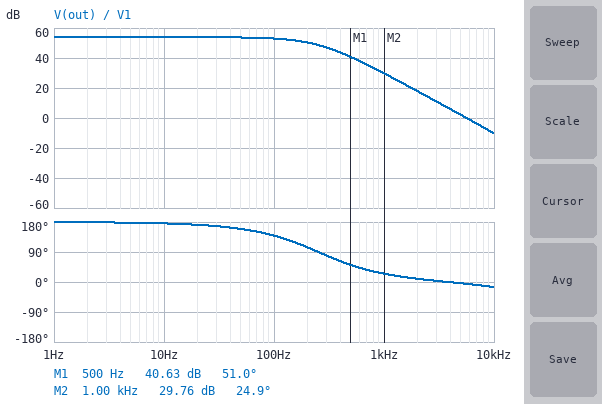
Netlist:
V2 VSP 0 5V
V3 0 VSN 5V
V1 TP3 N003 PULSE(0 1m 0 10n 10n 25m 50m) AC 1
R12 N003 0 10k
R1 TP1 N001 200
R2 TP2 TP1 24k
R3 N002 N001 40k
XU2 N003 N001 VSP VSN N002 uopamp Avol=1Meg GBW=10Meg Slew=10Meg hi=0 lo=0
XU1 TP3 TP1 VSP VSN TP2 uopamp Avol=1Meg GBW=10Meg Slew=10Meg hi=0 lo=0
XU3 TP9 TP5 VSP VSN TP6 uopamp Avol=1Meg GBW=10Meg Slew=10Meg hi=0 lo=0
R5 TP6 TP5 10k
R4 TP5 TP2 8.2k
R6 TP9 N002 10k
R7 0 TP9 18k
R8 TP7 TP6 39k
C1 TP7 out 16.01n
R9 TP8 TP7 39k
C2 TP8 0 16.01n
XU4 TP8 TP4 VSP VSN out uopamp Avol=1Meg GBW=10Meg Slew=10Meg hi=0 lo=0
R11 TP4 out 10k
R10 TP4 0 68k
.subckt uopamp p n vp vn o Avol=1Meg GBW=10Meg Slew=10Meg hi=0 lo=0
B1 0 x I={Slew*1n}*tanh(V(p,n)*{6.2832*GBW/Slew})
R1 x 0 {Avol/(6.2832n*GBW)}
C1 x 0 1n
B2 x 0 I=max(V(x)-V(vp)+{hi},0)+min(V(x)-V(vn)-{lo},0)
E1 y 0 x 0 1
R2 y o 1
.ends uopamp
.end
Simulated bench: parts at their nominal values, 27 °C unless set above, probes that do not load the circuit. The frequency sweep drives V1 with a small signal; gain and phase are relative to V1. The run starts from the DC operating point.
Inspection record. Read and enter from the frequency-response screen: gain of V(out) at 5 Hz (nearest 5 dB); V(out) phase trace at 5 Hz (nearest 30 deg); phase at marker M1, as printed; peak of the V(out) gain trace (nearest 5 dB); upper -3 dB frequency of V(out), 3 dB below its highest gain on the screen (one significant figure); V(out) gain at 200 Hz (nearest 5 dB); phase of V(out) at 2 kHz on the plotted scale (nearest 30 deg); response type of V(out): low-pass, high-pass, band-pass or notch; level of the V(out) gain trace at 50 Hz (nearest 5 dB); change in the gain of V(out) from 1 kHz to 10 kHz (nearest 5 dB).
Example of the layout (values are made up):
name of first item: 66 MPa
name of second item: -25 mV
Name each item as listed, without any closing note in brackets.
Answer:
gain of V(out) at 5 Hz: 55 dB
V(out) phase trace at 5 Hz: 180 deg
phase at marker M1, as printed: 51.0 deg
peak of the V(out) gain trace: 55 dB
upper -3 dB frequency of V(out), 3 dB below its highest gain on the screen: 200 Hz
V(out) gain at 200 Hz: 50 dB
phase of V(out) at 2 kHz on the plotted scale: 0 deg
response type of V(out): low-pass, high-pass, band-pass or notch: low-pass
level of the V(out) gain trace at 50 Hz: 55 dB
change in the gain of V(out) from 1 kHz to 10 kHz: -40 dB
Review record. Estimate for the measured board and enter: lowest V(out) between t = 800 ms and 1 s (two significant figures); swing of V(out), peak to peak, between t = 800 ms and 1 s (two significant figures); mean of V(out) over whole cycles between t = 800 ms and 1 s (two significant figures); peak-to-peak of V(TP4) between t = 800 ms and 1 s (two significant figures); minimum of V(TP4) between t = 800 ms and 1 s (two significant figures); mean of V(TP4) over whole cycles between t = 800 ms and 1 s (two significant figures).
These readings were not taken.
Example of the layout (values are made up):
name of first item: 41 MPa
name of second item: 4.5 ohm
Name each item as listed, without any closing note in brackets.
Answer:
lowest V(out) between t = 800 ms and 1 s: -500 mV
swing of V(out), peak to peak, between t = 800 ms and 1 s: 500 mV
mean of V(out) over whole cycles between t = 800 ms and 1 s: -250 mV
peak-to-peak of V(TP4) between t = 800 ms and 1 s: 430 mV
minimum of V(TP4) between t = 800 ms and 1 s: -430 mV
mean of V(TP4) over whole cycles between t = 800 ms and 1 s: -220 mV
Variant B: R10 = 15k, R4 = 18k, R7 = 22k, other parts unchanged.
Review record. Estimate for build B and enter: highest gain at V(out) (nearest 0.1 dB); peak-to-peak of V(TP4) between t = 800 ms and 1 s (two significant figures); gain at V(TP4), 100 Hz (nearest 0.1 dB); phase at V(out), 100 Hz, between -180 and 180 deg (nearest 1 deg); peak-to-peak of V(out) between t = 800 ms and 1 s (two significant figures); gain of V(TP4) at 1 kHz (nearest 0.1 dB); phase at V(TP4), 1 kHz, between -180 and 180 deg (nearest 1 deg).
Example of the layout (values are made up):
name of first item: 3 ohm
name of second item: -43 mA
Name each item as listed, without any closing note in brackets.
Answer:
highest gain at V(out): 53.5 dB
peak-to-peak of V(TP4) between t = 800 ms and 1 s: 320 mV
gain at V(TP4), 100 Hz: 49.0 dB
phase at V(out), 100 Hz, between -180 and 180 deg: 148 deg
peak-to-peak of V(out) between t = 800 ms and 1 s: 530 mV
gain of V(TP4) at 1 kHz: 25.3 dB
phase at V(TP4), 1 kHz, between -180 and 180 deg: 18 deg
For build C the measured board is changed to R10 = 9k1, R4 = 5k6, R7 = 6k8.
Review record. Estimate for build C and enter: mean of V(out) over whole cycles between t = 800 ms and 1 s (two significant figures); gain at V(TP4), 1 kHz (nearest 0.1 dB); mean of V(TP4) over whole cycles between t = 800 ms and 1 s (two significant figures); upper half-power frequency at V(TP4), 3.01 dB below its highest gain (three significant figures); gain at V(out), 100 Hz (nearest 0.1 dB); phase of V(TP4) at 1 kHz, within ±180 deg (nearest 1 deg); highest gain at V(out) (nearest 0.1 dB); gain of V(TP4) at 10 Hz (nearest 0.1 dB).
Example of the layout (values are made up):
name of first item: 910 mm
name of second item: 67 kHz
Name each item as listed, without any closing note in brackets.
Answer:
mean of V(out) over whole cycles between t = 800 ms and 1 s: -460 mV
gain at V(TP4), 1 kHz: 29.5 dB
mean of V(TP4) over whole cycles between t = 800 ms and 1 s: -220 mV
upper half-power frequency at V(TP4), 3.01 dB below its highest gain: 301 Hz
gain at V(out), 100 Hz: 60.1 dB
phase of V(TP4) at 1 kHz, within ±180 deg: 12 deg
highest gain at V(out): 61.2 dB
gain of V(TP4) at 10 Hz: 52.9 dB
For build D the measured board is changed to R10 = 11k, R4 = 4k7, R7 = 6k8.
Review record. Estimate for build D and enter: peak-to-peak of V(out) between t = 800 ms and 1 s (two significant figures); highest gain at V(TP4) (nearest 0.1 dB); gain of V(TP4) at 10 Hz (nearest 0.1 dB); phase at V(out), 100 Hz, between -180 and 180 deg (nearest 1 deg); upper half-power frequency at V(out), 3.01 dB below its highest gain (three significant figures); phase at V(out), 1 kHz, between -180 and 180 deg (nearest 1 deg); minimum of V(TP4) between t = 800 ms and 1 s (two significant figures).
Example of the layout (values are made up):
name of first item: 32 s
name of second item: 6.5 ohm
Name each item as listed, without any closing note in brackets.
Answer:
peak-to-peak of V(out) between t = 800 ms and 1 s: 1.2 V
highest gain at V(TP4): 54.9 dB
gain of V(TP4) at 10 Hz: 54.2 dB
phase at V(out), 100 Hz, between -180 and 180 deg: 153 deg
upper half-power frequency at V(out), 3.01 dB below its highest gain: 293 Hz
phase at V(out), 1 kHz, between -180 and 180 deg: 15 deg
minimum of V(TP4) between t = 800 ms and 1 s: -580 mV
